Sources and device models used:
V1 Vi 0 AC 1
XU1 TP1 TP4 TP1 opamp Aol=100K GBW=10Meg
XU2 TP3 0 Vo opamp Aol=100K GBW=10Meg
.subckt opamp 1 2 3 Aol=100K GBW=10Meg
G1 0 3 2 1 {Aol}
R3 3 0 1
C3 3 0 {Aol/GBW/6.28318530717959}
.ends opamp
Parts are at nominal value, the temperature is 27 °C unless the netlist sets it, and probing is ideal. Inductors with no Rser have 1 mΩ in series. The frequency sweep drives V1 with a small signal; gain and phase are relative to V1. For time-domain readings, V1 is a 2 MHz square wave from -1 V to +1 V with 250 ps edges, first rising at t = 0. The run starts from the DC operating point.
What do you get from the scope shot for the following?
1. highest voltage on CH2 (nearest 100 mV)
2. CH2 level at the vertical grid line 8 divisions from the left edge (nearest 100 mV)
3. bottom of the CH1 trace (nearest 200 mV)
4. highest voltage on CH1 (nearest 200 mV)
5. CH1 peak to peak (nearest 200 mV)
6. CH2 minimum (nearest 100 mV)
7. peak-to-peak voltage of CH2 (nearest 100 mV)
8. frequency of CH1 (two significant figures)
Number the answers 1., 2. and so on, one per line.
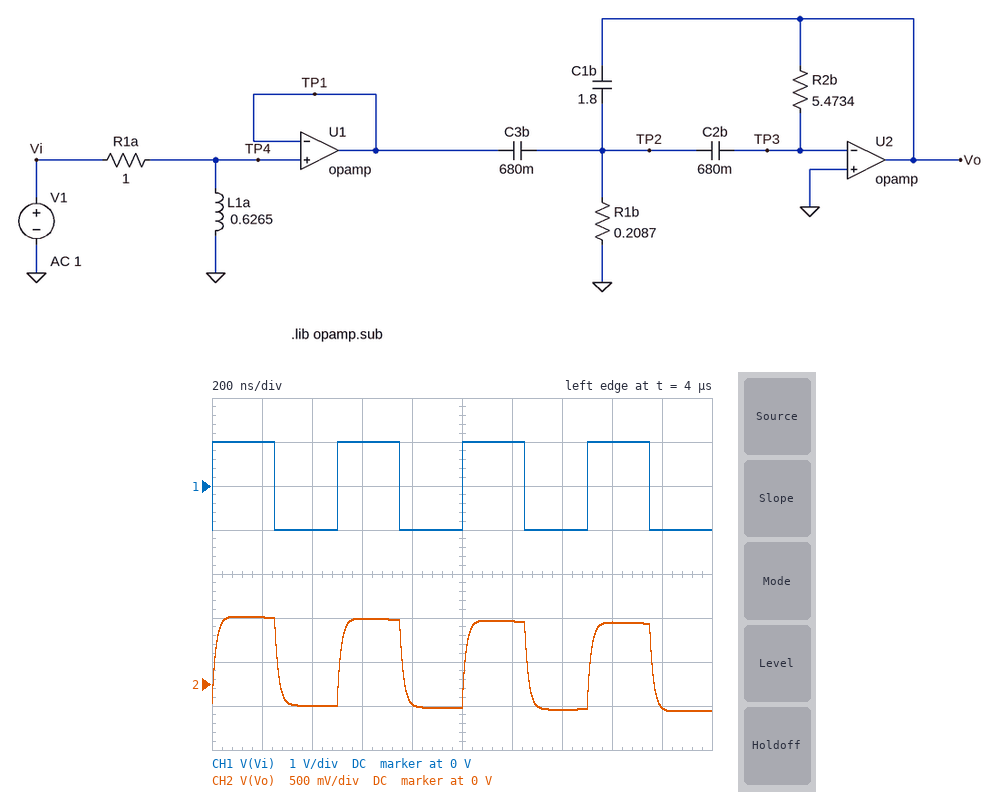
1. 800 mV
2. 700 mV
3. -1.0 V
4. 1.0 V
5. 2.0 V
6. -300 mV
7. 1.1 V
8. 2.0 MHz
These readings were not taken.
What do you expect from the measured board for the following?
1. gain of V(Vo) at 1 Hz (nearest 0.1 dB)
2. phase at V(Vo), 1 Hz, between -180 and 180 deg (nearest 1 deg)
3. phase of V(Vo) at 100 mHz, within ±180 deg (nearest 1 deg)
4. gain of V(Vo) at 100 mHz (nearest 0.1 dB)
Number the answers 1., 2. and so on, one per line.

1. -8.6 dB
2. -161 deg
3. 26 deg
4. -18.1 dB
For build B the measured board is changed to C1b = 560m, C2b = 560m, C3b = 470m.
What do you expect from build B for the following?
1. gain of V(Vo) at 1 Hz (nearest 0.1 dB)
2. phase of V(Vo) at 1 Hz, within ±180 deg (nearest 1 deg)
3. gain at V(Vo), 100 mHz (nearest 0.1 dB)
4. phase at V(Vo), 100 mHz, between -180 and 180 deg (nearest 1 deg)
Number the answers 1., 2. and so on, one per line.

1. -1.3 dB
2. -157 deg
3. -26.2 dB
4. 55 deg
